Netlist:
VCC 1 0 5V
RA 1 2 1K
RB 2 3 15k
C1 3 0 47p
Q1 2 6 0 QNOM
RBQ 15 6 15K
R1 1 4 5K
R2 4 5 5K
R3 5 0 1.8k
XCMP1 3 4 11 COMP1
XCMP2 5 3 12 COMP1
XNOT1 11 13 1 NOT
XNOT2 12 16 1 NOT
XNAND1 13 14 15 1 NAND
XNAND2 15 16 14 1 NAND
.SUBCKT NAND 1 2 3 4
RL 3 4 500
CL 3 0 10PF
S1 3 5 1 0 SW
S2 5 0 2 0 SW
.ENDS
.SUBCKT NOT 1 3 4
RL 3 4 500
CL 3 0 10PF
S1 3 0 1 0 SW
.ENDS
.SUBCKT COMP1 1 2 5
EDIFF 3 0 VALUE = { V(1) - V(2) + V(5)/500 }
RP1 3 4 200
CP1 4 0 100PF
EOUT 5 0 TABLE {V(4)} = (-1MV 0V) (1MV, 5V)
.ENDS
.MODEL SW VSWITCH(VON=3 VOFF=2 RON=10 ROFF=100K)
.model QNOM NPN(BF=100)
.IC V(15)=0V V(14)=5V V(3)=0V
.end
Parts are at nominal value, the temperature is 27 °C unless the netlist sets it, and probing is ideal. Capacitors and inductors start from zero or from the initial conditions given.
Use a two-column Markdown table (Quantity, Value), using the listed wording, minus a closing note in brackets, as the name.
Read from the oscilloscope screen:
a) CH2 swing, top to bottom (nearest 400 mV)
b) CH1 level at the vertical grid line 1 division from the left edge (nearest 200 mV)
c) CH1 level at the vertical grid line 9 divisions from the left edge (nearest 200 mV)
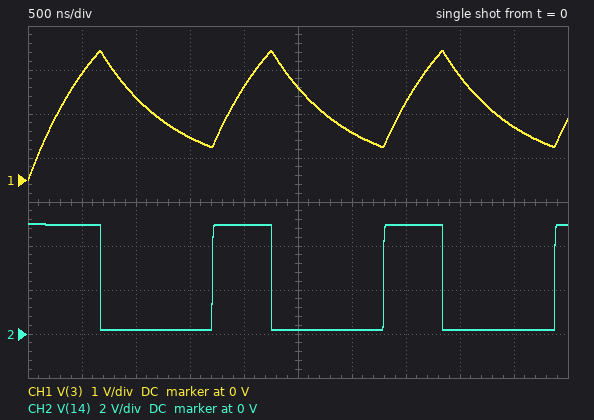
| Quantity | Value |
|---|---|
| CH2 swing, top to bottom | 4.8 V |
| CH1 level at the vertical grid line 1 division from the left edge | 2.4 V |
| CH1 level at the vertical grid line 9 divisions from the left edge | 1.2 V |
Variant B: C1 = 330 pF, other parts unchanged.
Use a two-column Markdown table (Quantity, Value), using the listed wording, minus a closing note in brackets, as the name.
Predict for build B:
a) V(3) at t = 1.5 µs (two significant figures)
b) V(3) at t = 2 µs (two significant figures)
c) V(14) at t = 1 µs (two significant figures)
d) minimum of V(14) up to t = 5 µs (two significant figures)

| Quantity | Value |
|---|---|
| V(3) at t = 1.5 µs | 1.2 V |
| V(3) at t = 2 µs | 1.6 V |
| V(14) at t = 1 µs | 5.0 V |
| minimum of V(14) up to t = 5 µs | 190 mV |
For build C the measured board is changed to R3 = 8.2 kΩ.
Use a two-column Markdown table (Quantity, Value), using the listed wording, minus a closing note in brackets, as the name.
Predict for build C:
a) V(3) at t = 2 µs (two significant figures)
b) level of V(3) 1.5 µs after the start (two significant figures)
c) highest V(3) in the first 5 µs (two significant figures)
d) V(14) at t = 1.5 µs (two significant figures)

| Quantity | Value |
|---|---|
| V(3) at t = 2 µs | 3.4 V |
| level of V(3) 1.5 µs after the start | 2.6 V |
| highest V(3) in the first 5 µs | 3.7 V |
| V(14) at t = 1.5 µs | 5.0 V |
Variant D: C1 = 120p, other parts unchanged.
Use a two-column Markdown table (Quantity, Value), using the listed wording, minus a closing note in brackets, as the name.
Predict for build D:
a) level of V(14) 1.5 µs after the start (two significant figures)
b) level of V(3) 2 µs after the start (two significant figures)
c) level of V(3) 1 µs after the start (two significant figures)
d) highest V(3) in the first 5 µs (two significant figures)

| Quantity | Value |
|---|---|
| level of V(14) 1.5 µs after the start | 5.0 V |
| level of V(3) 2 µs after the start | 2.4 V |
| level of V(3) 1 µs after the start | 2.0 V |
| highest V(3) in the first 5 µs | 2.9 V |
